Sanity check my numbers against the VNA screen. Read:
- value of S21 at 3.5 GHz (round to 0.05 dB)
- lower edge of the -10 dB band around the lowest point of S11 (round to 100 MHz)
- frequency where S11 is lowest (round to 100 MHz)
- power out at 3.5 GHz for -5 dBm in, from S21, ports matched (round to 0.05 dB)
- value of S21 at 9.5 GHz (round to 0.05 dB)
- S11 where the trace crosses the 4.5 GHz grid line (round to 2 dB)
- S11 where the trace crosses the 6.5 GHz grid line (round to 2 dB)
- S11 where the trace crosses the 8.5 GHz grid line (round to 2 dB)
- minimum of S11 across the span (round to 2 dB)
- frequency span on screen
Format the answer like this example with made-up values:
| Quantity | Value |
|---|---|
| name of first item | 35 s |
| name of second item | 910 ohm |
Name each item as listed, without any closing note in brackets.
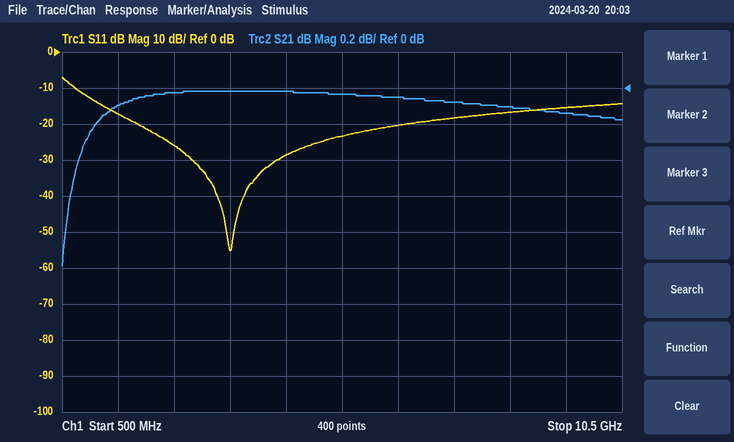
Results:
| Quantity | Value |
|---|---|
| value of S21 at 3.5 GHz | 0.00 dB |
| lower edge of the -10 dB band around the lowest point of S11 | 700 MHz |
| frequency where S11 is lowest | 3.5 GHz |
| power out at 3.5 GHz for -5 dBm in, from S21, ports matched | -5.00 dBm |
| value of S21 at 9.5 GHz | -0.15 dB |
| S11 where the trace crosses the 4.5 GHz grid line | -28 dB |
| S11 where the trace crosses the 6.5 GHz grid line | -20 dB |
| S11 where the trace crosses the 8.5 GHz grid line | -16 dB |
| minimum of S11 across the span | -56 dB |
| frequency span on screen | 10 GHz |
